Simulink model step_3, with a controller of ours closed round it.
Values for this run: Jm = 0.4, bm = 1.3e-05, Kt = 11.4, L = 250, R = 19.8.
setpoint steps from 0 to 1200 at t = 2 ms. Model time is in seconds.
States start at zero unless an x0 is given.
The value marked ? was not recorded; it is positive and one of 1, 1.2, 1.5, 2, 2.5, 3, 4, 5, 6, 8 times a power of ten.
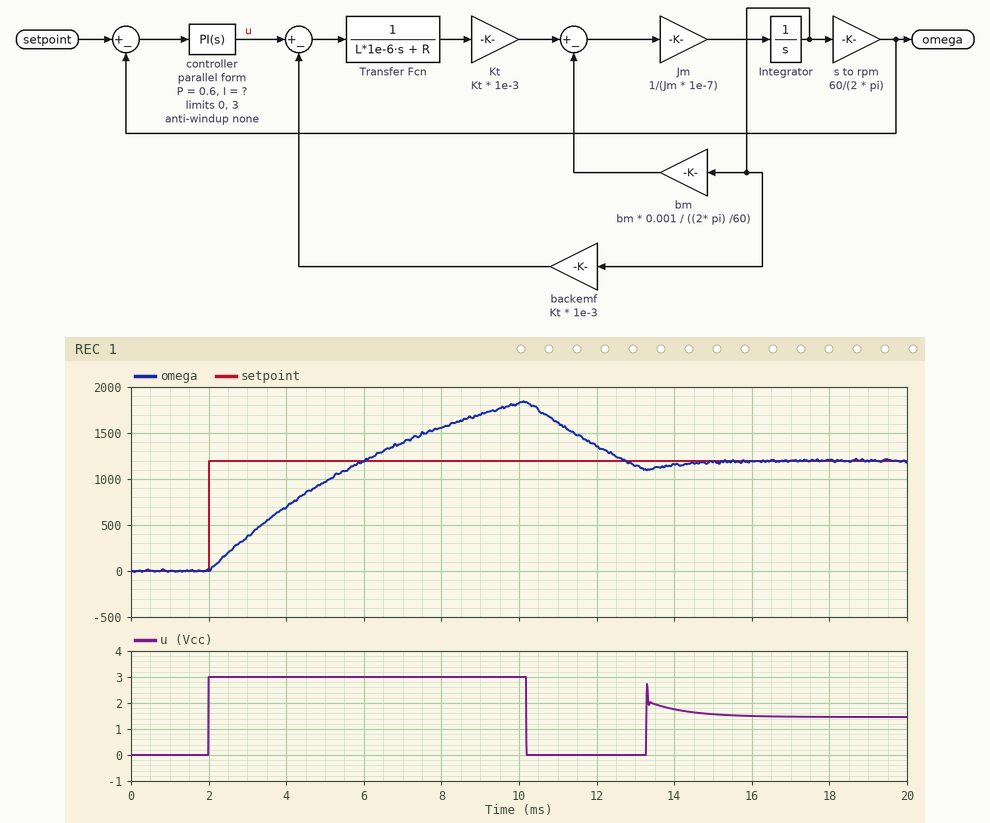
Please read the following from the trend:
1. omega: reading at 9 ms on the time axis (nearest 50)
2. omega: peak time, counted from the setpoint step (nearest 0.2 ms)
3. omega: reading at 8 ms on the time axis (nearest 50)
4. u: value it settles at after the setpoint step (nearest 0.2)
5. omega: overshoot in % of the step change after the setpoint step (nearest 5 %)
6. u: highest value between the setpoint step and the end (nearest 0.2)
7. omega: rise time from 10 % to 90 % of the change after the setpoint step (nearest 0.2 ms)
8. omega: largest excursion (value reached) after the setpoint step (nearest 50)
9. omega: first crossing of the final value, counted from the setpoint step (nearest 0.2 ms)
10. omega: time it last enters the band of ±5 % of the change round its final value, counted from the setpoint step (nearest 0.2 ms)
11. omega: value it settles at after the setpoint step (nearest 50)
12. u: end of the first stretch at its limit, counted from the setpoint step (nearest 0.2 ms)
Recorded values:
1700
8.2 ms
1550
1.4
55 %
3.0
3.2 ms
1850
4.0 ms
11.8 ms
1200
8.2 ms
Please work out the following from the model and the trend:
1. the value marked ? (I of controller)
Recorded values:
600
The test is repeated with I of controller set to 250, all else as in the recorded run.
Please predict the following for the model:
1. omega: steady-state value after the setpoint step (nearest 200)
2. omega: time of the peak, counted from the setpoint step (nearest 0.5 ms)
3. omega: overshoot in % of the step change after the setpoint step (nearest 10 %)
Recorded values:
1200
7.0 ms
40 %
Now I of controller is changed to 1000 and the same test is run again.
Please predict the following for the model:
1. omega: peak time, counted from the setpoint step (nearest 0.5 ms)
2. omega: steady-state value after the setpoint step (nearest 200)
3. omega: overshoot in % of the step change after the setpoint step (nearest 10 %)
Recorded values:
8.5 ms
1200
60 %
